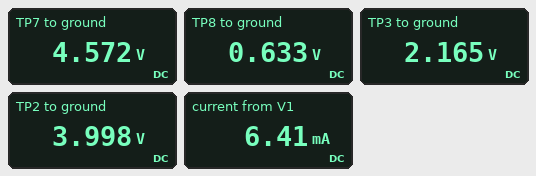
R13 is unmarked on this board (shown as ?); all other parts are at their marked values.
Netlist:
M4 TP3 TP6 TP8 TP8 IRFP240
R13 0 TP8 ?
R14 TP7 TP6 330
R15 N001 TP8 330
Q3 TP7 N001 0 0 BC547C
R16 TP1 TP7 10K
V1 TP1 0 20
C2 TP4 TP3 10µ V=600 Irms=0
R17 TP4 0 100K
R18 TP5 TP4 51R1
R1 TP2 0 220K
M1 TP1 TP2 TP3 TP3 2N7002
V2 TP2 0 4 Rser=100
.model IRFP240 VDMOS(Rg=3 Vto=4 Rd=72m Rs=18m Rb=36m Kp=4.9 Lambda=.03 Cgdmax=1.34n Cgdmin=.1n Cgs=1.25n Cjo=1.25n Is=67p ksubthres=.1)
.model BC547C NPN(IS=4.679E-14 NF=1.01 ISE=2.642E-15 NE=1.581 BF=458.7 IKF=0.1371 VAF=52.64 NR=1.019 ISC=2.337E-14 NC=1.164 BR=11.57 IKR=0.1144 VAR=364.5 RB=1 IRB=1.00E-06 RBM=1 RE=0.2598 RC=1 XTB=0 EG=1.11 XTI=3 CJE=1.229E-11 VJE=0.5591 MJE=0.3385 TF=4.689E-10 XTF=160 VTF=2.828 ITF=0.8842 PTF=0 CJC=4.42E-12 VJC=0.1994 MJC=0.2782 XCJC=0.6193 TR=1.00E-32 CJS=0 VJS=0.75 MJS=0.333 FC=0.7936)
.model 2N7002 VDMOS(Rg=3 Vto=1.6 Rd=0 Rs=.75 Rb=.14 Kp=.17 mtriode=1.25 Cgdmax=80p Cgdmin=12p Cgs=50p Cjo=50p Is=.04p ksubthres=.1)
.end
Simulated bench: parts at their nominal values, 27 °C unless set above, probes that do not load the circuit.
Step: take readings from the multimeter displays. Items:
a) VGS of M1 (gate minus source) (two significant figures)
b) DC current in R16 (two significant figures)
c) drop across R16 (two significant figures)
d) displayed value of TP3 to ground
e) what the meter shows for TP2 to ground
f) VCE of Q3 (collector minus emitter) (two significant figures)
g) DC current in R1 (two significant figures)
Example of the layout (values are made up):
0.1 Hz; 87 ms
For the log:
1.8 V; 1.5 mA; 15 V; 2.165 V; 3.998 V; 4.6 V; 18 µA
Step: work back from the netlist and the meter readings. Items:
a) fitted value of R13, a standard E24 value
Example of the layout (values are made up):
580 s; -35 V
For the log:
130 Ω
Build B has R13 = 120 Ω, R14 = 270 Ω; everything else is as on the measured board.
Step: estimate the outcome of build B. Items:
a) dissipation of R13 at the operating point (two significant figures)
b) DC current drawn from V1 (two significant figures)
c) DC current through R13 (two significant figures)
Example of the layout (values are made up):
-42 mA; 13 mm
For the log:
3.3 mW; 6.8 mA; 5.3 mA
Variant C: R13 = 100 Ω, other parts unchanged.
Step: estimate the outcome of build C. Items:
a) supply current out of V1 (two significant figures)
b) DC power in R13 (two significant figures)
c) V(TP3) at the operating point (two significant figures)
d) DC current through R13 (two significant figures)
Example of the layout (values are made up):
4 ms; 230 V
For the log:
7.9 mA; 4.0 mW; 2.1 V; 6.3 mA
